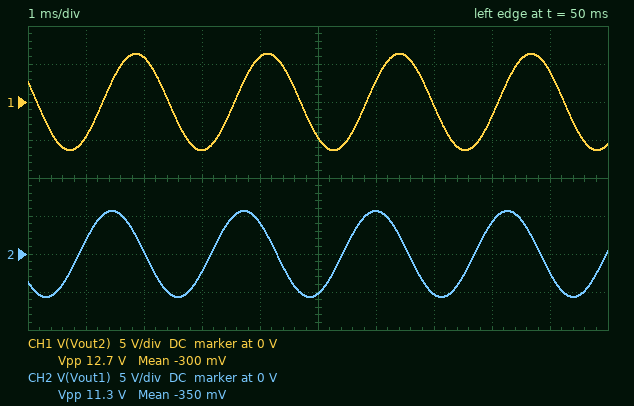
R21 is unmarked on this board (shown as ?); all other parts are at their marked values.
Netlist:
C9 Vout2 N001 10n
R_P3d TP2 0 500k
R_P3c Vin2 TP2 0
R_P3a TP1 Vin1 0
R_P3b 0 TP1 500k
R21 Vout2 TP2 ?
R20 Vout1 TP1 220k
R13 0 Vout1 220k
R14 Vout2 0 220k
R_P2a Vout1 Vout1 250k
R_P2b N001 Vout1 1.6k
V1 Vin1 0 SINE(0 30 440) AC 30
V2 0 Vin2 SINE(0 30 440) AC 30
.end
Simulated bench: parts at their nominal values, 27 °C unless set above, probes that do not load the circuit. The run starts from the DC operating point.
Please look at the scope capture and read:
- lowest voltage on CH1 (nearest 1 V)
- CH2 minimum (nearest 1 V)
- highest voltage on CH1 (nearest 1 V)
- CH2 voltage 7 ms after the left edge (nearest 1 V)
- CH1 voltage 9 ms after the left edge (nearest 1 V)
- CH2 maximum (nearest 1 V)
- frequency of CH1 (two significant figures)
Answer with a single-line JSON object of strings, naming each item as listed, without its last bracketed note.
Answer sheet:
{"lowest voltage on CH1": "-6 V", "CH2 minimum": "-6 V", "highest voltage on CH1": "6 V", "CH2 voltage 7 ms after the left edge": "-5 V", "CH1 voltage 9 ms after the left edge": "4 V", "CH2 maximum": "6 V", "frequency of CH1": "440 Hz"}
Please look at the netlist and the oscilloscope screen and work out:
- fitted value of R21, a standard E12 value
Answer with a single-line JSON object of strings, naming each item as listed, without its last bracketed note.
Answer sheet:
{"fitted value of R21, a standard E12 value": "120 kΩ"}
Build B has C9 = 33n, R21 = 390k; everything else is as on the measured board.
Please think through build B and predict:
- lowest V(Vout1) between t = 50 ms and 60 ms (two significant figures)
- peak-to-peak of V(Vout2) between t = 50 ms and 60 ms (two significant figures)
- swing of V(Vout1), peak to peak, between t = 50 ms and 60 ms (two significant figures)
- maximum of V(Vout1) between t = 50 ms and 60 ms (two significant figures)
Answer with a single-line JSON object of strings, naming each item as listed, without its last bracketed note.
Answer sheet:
{"lowest V(Vout1) between t = 50 ms and 60 ms": "-3.8 V", "peak-to-peak of V(Vout2) between t = 50 ms and 60 ms": "7.2 V", "swing of V(Vout1), peak to peak, between t = 50 ms and 60 ms": "7.6 V", "maximum of V(Vout1) between t = 50 ms and 60 ms": "3.8 V"}
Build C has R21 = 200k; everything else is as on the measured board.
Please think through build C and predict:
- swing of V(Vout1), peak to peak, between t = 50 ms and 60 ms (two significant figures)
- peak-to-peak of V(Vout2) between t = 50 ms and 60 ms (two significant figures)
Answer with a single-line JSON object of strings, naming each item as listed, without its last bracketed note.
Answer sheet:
{"swing of V(Vout1), peak to peak, between t = 50 ms and 60 ms": "5.1 V", "peak-to-peak of V(Vout2) between t = 50 ms and 60 ms": "5.4 V"}
